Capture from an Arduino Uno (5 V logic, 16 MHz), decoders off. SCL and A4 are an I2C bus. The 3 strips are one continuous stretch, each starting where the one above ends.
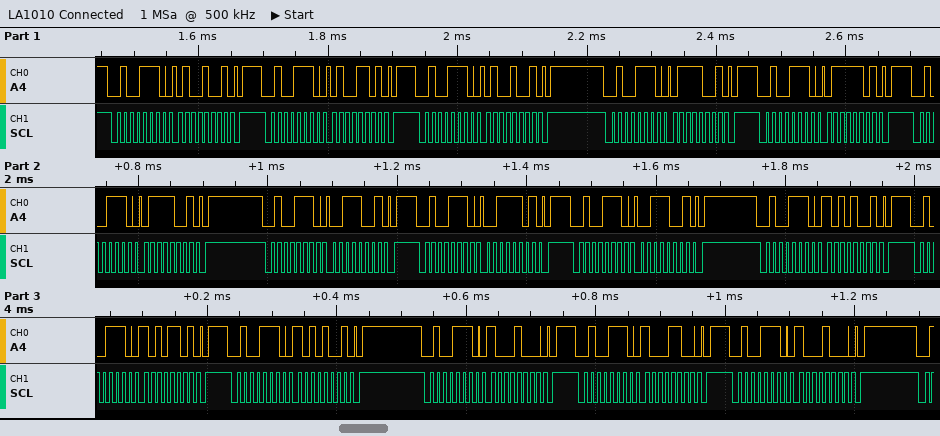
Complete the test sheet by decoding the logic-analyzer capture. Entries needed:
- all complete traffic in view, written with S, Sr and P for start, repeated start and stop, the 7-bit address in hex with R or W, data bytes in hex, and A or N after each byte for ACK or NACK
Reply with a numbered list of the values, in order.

1. S 27W A 49 A P S 27W A 4D A P S 27W A 49 A P S 27W A 79 A P S 27W A 7D A P S 27W A 79 A P S 27W A 39 A P S 27W A 3D A P S 27W A 39 A P S 27W A A9 A P S 27W A AD A P S 27W A A9 A P S 27W A 88 A P S 27W A 8C A P S 27W A 88 A P
